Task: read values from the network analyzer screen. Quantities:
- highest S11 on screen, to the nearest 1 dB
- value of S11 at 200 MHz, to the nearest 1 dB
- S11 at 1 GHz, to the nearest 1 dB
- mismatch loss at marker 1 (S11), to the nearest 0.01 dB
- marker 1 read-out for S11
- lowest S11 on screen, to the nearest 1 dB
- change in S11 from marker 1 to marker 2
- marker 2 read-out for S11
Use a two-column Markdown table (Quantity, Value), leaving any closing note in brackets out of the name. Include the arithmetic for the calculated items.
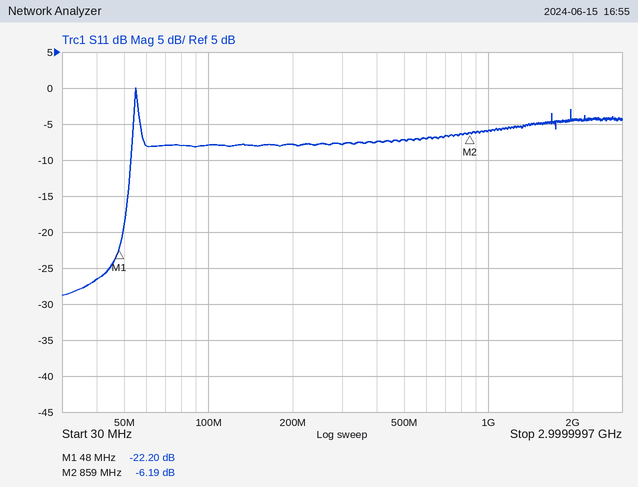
| Quantity | Value |
|---|---|
| highest S11 on screen, to the nearest 1 dB | 0 dB |
| value of S11 at 200 MHz, to the nearest 1 dB | -8 dB |
| S11 at 1 GHz, to the nearest 1 dB | -6 dB |
| mismatch loss at marker 1 (S11), to the nearest 0.01 dB | −10 log10(1 − 10^(-22.2/10)) ≈ 0.03 dB |
| marker 1 read-out for S11 | -22.20 dB |
| lowest S11 on screen, to the nearest 1 dB | -29 dB |
| change in S11 from marker 1 to marker 2 | -6.19 − (-22.2) = 16.01 dB |
| marker 2 read-out for S11 | -6.19 dB |
